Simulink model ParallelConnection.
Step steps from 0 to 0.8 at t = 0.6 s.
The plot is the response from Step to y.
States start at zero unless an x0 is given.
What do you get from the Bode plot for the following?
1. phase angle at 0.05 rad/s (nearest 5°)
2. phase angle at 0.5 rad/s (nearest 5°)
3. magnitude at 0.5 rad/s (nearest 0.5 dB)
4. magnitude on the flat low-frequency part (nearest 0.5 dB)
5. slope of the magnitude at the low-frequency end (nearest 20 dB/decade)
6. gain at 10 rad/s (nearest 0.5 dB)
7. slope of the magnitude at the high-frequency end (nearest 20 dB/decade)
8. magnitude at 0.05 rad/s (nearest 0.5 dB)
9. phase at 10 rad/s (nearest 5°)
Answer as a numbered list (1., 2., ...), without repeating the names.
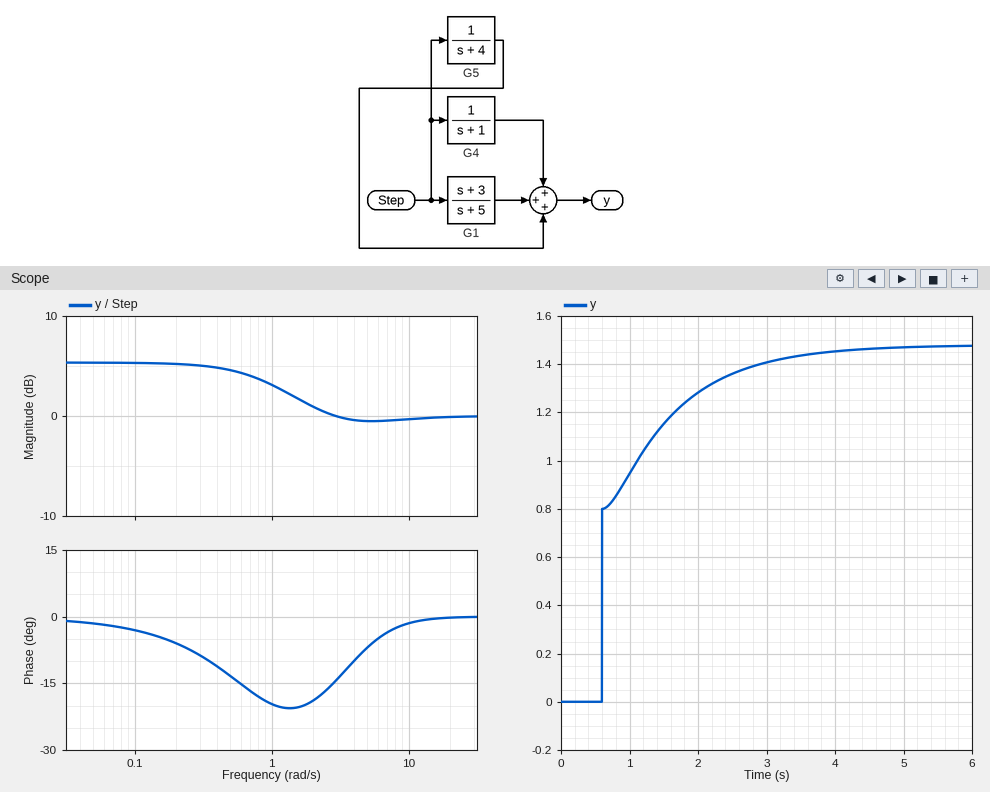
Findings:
1. 0°
2. -15°
3. 4.5 dB
4. 5.5 dB
5. 0 dB/decade
6. -0.5 dB
7. 0 dB/decade
8. 5.5 dB
9. 0°
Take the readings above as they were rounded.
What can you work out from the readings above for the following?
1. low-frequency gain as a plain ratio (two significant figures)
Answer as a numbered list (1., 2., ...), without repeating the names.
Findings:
1. 1.9
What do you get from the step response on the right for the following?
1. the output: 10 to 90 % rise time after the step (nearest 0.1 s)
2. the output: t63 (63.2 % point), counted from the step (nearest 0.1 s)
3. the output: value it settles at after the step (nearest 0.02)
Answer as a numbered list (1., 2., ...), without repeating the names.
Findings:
1. 1.7 s
2. 0.4 s
3. 1.48
